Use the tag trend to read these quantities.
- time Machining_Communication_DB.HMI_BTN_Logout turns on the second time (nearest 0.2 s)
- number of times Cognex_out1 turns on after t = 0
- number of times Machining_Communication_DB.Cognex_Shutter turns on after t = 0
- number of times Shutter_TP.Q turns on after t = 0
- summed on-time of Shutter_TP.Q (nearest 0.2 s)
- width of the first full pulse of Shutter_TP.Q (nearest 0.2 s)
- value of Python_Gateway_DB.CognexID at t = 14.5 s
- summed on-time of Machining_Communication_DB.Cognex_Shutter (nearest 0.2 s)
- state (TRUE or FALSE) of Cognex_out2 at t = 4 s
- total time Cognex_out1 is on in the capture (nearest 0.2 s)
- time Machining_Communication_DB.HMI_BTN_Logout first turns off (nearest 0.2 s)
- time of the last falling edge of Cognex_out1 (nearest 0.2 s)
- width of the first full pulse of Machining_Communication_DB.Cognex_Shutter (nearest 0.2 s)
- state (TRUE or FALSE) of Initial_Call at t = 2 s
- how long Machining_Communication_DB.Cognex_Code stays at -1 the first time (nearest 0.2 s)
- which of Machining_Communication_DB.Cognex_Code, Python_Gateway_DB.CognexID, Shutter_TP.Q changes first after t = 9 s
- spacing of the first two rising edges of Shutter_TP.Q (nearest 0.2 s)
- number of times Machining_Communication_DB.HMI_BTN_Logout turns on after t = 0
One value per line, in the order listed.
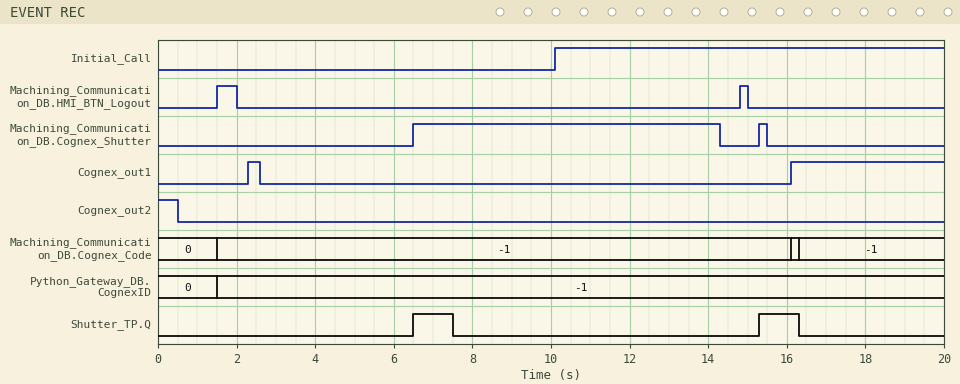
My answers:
14.8 s
2
2
2
2.0 s
1.0 s
-1
8.0 s
FALSE
4.2 s
2.0 s
2.6 s
7.8 s
FALSE
14.6 s
Shutter_TP.Q
8.8 s
2
